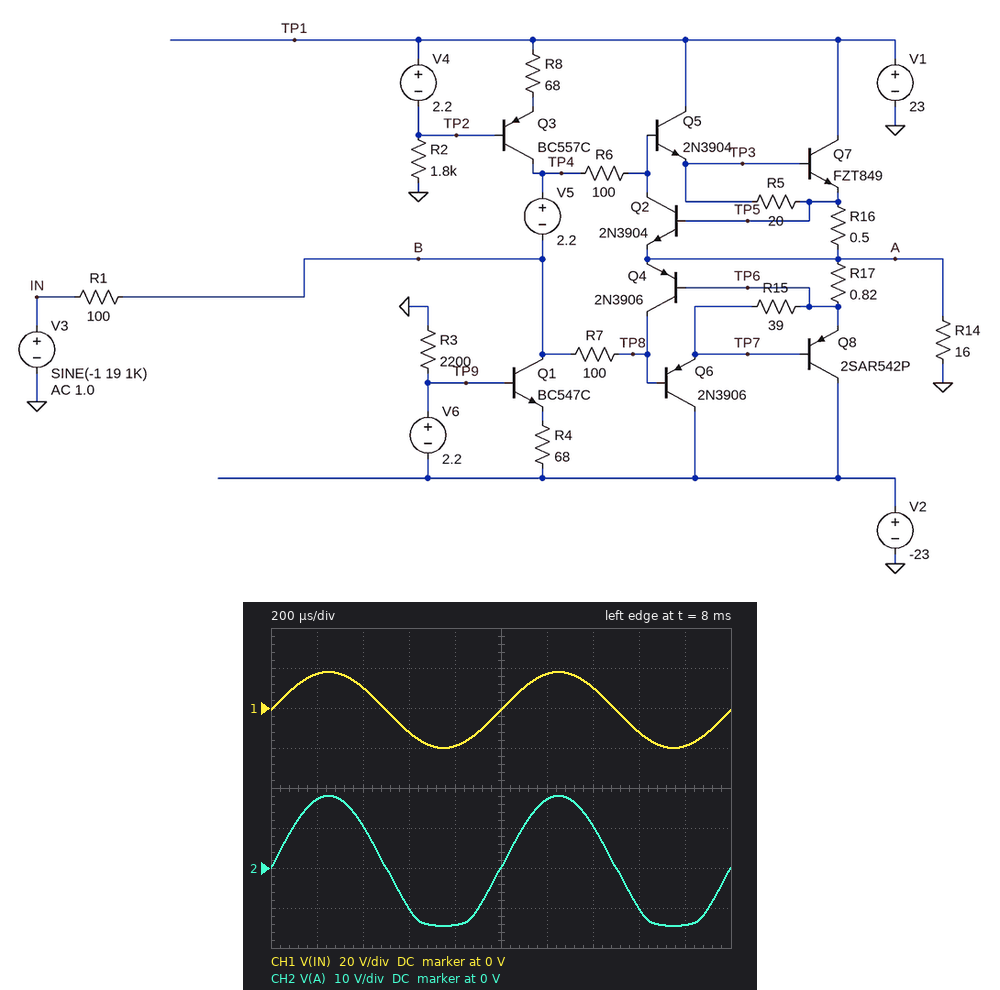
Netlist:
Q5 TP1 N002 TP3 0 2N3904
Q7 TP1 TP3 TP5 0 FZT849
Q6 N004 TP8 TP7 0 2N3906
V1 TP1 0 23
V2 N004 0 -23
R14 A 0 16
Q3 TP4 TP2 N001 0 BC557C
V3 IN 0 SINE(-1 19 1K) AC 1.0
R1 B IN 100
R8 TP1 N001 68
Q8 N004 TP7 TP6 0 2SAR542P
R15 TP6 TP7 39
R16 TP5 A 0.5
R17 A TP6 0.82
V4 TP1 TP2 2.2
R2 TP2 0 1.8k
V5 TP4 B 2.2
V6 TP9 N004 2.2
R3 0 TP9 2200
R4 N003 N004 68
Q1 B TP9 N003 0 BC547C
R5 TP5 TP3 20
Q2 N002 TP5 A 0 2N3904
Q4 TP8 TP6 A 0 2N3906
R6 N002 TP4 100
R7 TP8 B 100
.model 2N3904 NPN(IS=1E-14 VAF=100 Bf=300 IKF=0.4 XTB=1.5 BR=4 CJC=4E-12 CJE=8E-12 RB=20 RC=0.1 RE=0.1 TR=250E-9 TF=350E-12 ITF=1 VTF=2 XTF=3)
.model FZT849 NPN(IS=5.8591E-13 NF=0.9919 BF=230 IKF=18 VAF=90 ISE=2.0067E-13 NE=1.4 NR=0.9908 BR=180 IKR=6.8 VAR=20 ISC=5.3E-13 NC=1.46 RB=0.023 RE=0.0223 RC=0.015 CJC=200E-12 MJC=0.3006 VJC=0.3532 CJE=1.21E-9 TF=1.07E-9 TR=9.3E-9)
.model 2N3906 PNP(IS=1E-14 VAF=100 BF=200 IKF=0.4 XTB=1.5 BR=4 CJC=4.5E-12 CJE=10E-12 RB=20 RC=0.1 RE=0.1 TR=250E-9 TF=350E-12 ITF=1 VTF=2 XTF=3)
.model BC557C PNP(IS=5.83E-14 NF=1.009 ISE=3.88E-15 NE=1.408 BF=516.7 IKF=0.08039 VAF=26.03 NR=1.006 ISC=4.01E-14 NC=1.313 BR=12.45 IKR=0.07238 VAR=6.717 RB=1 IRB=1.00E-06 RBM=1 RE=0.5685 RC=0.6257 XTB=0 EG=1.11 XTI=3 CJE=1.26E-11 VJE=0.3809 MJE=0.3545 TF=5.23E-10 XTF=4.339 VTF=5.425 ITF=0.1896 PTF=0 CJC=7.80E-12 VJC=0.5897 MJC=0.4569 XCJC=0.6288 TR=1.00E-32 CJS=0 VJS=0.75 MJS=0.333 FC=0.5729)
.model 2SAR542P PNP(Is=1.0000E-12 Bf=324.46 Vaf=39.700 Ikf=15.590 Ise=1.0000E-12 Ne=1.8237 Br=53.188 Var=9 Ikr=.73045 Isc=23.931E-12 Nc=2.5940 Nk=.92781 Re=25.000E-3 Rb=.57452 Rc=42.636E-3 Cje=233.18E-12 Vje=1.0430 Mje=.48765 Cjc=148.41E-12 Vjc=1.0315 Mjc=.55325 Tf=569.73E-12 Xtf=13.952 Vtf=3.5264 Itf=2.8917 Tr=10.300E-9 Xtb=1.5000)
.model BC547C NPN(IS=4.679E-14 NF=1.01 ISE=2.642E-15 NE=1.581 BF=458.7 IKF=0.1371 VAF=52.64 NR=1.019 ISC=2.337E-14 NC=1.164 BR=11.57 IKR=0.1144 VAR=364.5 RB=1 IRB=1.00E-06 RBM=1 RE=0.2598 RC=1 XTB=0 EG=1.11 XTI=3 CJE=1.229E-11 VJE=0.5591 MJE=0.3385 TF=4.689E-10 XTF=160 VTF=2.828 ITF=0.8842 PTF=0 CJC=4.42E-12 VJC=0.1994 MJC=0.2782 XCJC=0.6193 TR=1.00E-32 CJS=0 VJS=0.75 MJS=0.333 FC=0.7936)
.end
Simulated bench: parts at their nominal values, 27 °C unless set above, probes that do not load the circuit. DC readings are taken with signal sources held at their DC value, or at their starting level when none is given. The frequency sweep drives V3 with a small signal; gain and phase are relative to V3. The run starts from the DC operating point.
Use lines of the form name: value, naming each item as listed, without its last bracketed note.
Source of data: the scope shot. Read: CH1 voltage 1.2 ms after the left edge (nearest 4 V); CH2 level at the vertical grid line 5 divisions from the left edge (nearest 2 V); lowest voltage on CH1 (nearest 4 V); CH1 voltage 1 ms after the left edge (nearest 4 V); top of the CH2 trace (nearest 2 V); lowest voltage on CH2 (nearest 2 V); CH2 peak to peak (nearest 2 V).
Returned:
CH1 voltage 1.2 ms after the left edge: 16 V
CH2 level at the vertical grid line 5 divisions from the left edge: 0 V
lowest voltage on CH1: -20 V
CH1 voltage 1 ms after the left edge: 0 V
top of the CH2 trace: 18 V
lowest voltage on CH2: -14 V
CH2 peak to peak: 32 V
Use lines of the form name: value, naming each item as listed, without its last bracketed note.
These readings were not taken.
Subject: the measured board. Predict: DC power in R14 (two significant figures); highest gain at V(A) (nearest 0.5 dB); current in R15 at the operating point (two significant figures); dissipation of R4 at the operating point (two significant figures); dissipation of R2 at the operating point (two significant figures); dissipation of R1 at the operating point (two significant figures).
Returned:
DC power in R14: 860 µW
highest gain at V(A): -2.0 dB
current in R15 at the operating point: 10 mA
dissipation of R4 at the operating point: 33 mW
dissipation of R2 at the operating point: 240 mW
dissipation of R1 at the operating point: 230 nW
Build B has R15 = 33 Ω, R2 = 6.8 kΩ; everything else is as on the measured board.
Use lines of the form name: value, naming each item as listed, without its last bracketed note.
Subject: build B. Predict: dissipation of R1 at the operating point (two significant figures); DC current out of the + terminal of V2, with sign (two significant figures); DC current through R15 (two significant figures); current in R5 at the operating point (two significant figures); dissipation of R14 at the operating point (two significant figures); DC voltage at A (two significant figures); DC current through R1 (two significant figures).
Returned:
dissipation of R1 at the operating point: 270 nW
DC current out of the + terminal of V2, with sign: -43 mA
DC current through R15: 11 mA
current in R5 at the operating point: 18 mA
dissipation of R14 at the operating point: 700 µW
DC voltage at A: 110 mV
DC current through R1: 52 µA
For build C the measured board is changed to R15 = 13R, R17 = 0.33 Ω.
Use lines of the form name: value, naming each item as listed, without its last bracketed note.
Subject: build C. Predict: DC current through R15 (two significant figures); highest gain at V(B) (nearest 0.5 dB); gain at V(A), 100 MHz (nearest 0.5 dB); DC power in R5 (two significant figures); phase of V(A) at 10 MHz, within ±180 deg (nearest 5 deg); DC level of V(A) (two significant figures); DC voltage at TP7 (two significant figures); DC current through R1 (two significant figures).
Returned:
DC current through R15: 20 mA
highest gain at V(B): 0 dB
gain at V(A), 100 MHz: -10.0 dB
DC power in R5: 9.5 mW
phase of V(A) at 10 MHz, within ±180 deg: -5 deg
DC level of V(A): 22 mV
DC voltage at TP7: -250 mV
DC current through R1: 80 µA
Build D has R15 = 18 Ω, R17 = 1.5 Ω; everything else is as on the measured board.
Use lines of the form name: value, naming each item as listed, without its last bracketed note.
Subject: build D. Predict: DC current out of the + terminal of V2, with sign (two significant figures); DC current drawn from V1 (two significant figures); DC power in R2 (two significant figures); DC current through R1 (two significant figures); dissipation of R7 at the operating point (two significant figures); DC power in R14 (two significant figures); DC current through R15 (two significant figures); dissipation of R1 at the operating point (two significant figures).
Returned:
DC current out of the + terminal of V2, with sign: -48 mA
DC current drawn from V1: 54 mA
DC power in R2: 240 mW
DC current through R1: 67 µA
dissipation of R7 at the operating point: 480 nW
DC power in R14: 220 µW
DC current through R15: 16 mA
dissipation of R1 at the operating point: 450 nW
